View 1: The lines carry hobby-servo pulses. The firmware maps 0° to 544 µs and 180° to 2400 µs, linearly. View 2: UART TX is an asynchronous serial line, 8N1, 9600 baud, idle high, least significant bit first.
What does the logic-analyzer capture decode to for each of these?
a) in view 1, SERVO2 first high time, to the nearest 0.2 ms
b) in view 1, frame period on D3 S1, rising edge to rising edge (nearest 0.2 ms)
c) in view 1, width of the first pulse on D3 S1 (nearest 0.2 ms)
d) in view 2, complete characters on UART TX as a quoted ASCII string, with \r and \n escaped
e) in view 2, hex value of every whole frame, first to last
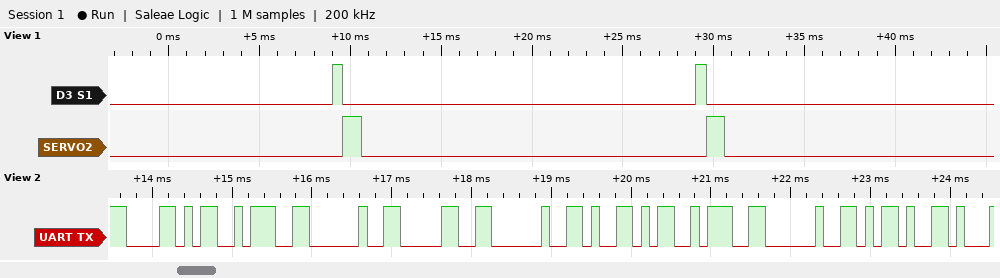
1.0 ms
20.0 ms
0.6 ms
"X: 0 Y: -"
58 3A 20 30 20 59 3A 20 2D
